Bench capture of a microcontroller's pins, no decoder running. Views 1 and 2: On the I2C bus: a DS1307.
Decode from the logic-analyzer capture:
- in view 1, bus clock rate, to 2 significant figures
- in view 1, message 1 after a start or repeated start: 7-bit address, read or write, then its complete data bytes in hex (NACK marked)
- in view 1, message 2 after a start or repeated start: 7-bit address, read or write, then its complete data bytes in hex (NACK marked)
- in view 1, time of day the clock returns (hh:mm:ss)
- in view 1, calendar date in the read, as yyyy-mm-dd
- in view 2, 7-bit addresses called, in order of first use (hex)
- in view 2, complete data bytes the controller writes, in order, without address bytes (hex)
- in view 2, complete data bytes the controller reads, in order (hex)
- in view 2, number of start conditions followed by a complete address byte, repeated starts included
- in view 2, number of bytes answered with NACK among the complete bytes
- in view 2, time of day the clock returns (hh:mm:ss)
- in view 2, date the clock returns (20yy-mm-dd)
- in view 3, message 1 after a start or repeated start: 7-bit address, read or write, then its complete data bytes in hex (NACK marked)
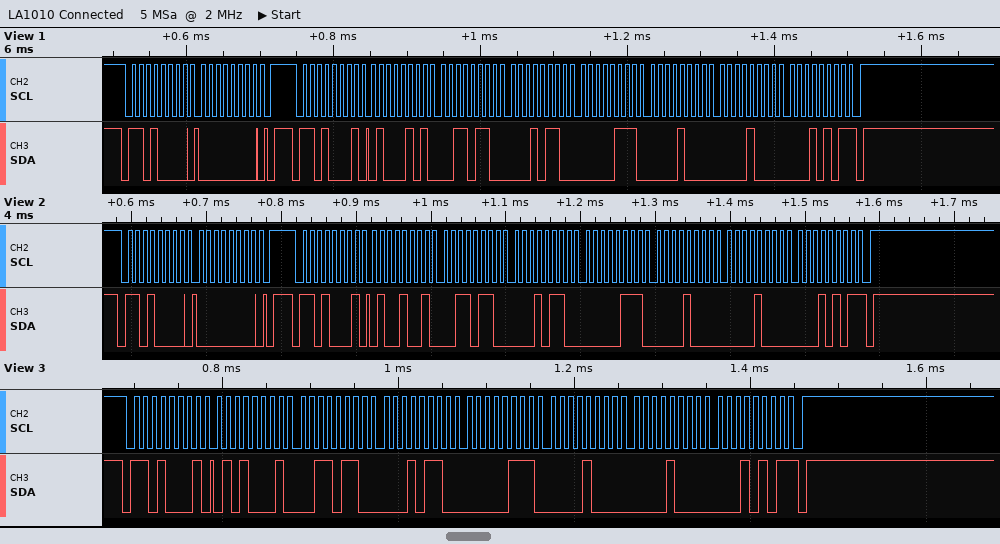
100 kHz
0x68 write: 00
0x68 read: 45 36 16 07 08 08 15 NACK
16:36:45
2015-08-08
0x68
00
49 36 16 07 08 08 15
2
1
16:36:49
2015-08-08
0x68 read: 51 36 16 07 08 08 15 NACK
